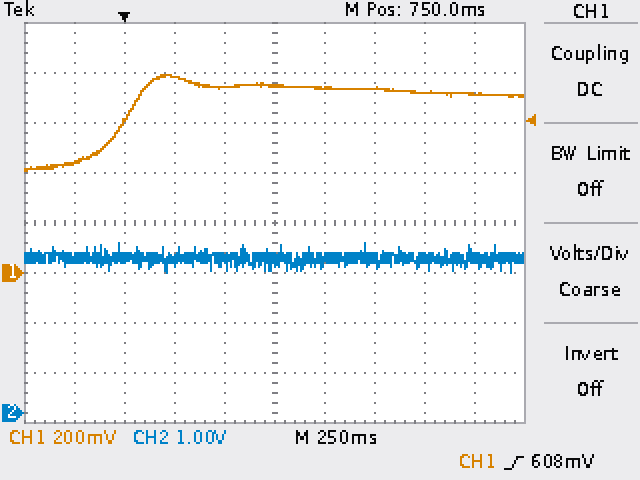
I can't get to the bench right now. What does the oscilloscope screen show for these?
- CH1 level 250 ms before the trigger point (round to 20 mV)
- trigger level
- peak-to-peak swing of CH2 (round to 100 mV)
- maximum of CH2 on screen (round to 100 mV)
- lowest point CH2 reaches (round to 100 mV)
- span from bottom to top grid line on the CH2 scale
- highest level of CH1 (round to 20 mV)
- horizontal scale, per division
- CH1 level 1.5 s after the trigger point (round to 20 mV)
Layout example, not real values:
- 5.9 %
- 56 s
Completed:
- 440 mV
- 608 mV
- 600 mV
- 3.4 V
- 2.8 V
- 8 V
- 800 mV
- 250 ms
- 720 mV
